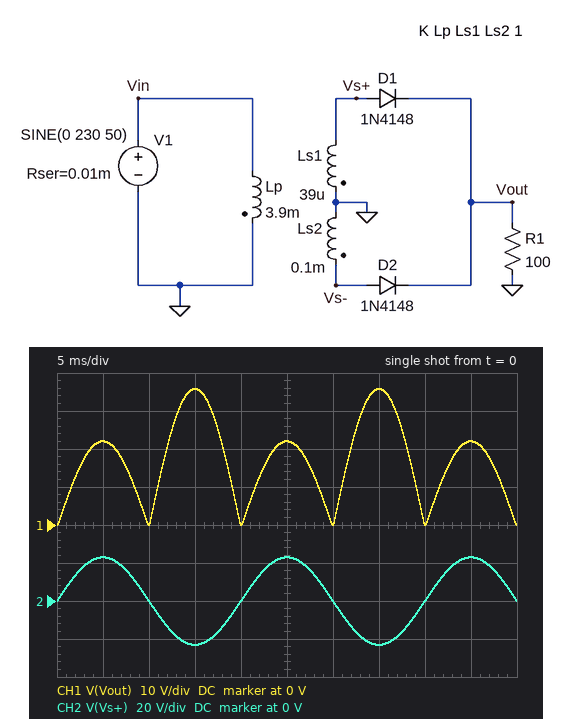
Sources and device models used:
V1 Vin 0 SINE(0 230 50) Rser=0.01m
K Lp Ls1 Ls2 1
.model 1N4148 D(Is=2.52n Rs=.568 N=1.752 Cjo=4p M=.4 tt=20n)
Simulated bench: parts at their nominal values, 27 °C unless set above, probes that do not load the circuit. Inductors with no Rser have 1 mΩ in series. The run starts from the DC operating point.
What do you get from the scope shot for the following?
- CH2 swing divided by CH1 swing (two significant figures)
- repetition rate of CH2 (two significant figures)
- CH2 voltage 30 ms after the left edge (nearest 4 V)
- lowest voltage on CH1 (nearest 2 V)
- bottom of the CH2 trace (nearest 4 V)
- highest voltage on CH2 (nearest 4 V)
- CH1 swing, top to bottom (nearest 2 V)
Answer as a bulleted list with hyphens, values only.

- 1.3
- 50 Hz
- 0 V
- 0 V
- -24 V
- 24 V
- 36 V
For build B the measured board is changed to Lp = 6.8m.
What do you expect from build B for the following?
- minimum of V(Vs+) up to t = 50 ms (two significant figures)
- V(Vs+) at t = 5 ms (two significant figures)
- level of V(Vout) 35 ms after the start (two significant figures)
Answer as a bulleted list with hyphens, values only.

- -17 V
- 17 V
- 27 V
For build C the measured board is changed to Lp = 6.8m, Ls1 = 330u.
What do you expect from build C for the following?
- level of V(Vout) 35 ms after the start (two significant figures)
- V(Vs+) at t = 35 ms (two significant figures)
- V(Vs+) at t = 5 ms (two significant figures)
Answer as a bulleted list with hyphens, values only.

- 27 V
- -51 V
- 51 V
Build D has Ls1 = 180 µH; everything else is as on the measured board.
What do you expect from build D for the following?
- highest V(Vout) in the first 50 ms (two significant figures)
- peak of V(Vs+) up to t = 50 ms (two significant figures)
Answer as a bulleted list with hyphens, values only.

- 48 V
- 49 V
